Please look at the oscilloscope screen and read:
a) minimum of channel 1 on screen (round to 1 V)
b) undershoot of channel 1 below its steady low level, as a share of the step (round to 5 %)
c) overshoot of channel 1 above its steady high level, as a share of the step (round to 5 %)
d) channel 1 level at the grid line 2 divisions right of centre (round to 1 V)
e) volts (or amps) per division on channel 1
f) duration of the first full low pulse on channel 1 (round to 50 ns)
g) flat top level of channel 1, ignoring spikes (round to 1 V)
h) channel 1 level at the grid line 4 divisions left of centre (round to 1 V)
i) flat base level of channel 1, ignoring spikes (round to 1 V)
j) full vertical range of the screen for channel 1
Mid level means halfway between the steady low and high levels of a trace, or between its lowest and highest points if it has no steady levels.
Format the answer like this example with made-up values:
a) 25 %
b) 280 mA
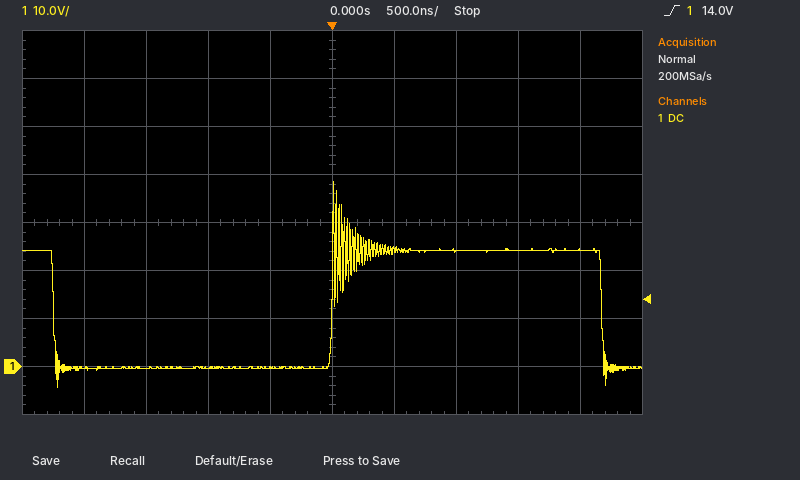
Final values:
a) -4 V
b) 15 %
c) 60 %
d) 24 V
e) 10 V
f) 2.25 µs
g) 24 V
h) 0 V
i) 0 V
j) 80 V
